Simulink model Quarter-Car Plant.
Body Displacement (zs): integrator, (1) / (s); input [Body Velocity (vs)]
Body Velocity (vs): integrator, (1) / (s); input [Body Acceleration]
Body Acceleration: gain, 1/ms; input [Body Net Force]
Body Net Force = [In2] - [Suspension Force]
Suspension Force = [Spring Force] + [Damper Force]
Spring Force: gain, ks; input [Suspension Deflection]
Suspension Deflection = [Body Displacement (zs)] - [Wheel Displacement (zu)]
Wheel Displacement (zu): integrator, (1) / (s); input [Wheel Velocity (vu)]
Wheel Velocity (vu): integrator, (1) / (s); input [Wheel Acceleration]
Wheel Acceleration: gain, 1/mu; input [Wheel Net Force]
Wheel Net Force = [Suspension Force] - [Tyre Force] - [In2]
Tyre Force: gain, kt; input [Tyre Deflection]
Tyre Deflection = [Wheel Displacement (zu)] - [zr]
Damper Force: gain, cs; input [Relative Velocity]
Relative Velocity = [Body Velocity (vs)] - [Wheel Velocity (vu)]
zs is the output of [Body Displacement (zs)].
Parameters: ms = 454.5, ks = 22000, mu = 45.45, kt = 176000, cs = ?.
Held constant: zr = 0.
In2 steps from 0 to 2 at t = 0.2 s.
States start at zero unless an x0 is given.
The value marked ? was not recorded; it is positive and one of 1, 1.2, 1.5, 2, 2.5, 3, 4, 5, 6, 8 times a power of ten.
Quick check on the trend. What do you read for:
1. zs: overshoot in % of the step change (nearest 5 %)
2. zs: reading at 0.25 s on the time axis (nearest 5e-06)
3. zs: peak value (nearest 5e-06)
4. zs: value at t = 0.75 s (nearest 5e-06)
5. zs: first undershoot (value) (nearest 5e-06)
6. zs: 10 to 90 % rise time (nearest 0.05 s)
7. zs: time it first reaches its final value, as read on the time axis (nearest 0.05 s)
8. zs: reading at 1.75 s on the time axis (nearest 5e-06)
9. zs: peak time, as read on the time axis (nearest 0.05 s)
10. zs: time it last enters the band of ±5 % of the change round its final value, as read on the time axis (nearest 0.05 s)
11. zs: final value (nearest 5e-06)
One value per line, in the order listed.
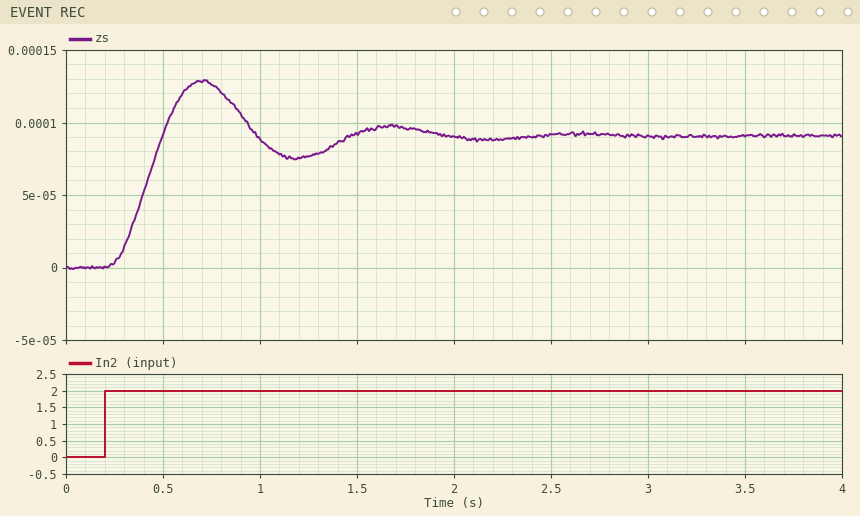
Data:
40 %
0.000005
0.000130
0.000125
0.000075
0.20 s
0.50 s
0.000095
0.70 s
1.80 s
0.000090
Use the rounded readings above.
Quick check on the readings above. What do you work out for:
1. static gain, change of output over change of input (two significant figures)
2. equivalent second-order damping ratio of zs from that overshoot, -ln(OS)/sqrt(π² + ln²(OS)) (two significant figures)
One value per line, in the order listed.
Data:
0.000045
0.28
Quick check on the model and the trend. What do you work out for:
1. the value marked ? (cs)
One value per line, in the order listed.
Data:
2000
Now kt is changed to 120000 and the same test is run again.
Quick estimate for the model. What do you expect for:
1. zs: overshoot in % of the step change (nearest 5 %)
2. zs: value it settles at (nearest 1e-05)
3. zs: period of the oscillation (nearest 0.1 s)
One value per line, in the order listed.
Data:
45 %
0.00009
1.0 s
